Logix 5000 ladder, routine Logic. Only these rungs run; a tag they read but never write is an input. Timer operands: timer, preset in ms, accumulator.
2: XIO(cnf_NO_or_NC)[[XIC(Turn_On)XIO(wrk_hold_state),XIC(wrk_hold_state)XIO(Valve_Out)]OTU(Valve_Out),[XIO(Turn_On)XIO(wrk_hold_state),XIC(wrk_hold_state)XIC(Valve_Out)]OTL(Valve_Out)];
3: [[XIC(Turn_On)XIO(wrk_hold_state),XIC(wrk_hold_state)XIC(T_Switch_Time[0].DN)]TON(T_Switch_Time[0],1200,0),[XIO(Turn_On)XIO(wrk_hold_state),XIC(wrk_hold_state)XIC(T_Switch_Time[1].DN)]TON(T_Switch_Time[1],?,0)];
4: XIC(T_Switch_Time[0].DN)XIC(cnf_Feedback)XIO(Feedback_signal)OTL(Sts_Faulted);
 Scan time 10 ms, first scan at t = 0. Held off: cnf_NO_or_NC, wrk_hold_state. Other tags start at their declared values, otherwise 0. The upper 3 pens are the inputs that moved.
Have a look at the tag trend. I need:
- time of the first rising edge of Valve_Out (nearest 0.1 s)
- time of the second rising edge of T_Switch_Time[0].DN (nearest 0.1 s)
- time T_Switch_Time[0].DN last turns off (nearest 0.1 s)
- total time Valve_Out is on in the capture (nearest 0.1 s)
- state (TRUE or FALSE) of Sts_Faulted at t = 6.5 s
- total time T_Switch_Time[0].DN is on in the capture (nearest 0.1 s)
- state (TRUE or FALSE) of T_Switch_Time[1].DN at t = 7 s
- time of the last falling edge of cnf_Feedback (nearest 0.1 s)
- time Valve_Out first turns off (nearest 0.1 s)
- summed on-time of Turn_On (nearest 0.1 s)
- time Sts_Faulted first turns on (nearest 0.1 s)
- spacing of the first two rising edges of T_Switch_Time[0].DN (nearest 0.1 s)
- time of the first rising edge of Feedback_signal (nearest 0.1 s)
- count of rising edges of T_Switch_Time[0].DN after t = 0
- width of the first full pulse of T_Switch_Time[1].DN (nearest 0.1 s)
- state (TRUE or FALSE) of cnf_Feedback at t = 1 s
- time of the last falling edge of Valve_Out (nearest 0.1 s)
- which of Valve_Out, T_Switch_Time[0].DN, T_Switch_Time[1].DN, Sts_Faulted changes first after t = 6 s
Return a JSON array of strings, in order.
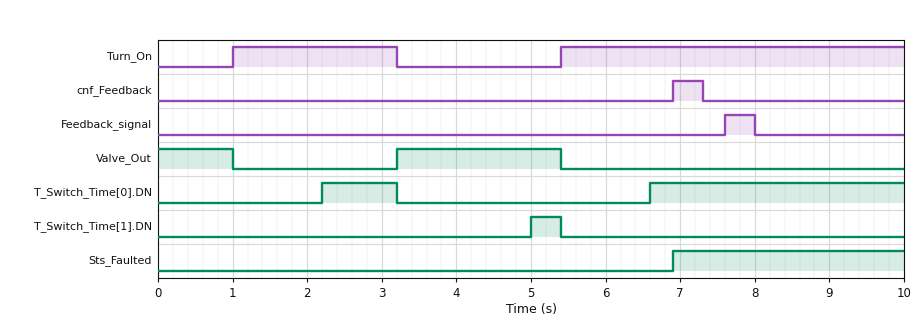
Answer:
["3.2 s", "6.6 s", "3.2 s", "3.2 s", "FALSE", "4.4 s", "FALSE", "7.3 s", "1.0 s", "6.8 s", "6.9 s", "4.4 s", "7.6 s", "2", "0.4 s", "FALSE", "5.4 s", "T_Switch_Time[0].DN"]
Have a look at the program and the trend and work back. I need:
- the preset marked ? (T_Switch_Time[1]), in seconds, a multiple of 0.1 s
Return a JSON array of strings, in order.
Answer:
["1.8 s"]
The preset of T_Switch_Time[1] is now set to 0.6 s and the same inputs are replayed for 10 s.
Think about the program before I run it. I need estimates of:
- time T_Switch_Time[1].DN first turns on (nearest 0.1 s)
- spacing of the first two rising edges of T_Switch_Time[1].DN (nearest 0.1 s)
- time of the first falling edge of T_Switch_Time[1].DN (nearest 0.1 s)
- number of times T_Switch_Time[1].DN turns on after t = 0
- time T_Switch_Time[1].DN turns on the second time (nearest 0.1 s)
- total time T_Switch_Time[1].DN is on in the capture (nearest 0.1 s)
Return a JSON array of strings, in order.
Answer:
["0.6 s", "3.2 s", "1.0 s", "2", "3.8 s", "2.0 s"]
